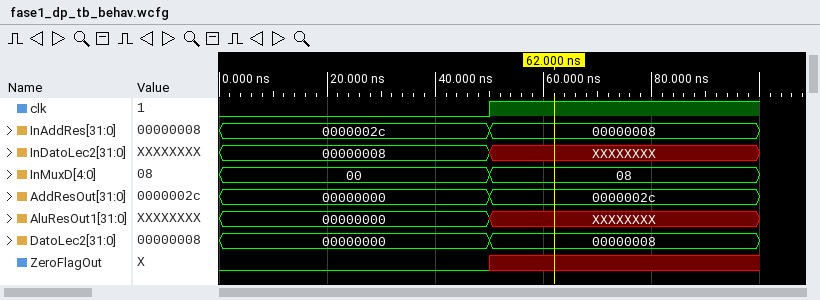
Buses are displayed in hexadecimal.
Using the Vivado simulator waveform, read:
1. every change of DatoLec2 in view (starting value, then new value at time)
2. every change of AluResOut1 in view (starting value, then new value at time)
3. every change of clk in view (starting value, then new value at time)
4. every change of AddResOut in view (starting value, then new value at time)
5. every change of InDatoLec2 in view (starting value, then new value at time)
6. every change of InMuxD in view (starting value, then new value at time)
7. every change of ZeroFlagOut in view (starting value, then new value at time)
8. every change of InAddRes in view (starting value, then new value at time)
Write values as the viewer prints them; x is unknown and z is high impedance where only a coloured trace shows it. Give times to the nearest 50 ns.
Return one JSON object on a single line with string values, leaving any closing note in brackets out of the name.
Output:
{"every change of DatoLec2 in view": "00000000, 00000008 at 50 ns", "every change of AluResOut1 in view": "00000000, XXXXXXXX at 50 ns", "every change of clk in view": "0, 1 at 50 ns", "every change of AddResOut in view": "00000000, 0000002c at 50 ns", "every change of InDatoLec2 in view": "00000008, XXXXXXXX at 50 ns", "every change of InMuxD in view": "00, 08 at 50 ns", "every change of ZeroFlagOut in view": "0, x at 50 ns", "every change of InAddRes in view": "0000002c, 00000008 at 50 ns"}
